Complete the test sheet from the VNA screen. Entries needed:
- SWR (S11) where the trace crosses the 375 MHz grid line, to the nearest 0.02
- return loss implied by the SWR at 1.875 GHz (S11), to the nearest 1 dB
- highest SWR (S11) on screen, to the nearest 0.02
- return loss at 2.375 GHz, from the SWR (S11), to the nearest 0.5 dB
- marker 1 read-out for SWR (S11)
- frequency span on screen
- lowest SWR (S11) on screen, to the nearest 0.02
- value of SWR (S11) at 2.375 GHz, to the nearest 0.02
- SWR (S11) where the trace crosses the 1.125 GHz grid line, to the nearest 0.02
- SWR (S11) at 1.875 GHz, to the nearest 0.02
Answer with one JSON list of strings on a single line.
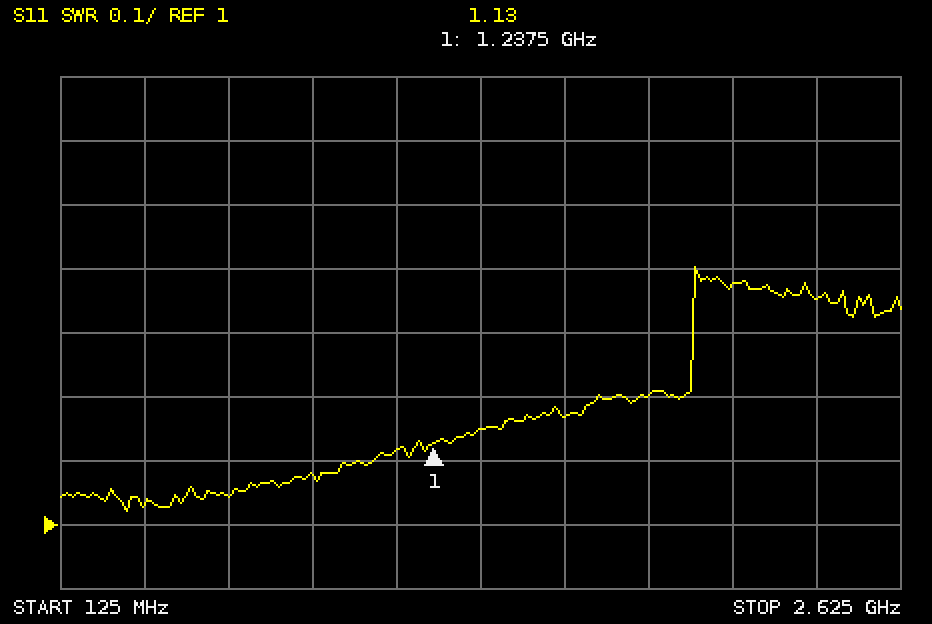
["1.04", "21 dB", "1.40", "16.5 dB", "1.13", "2.5 GHz", "1.02", "1.36", "1.12", "1.20"]
